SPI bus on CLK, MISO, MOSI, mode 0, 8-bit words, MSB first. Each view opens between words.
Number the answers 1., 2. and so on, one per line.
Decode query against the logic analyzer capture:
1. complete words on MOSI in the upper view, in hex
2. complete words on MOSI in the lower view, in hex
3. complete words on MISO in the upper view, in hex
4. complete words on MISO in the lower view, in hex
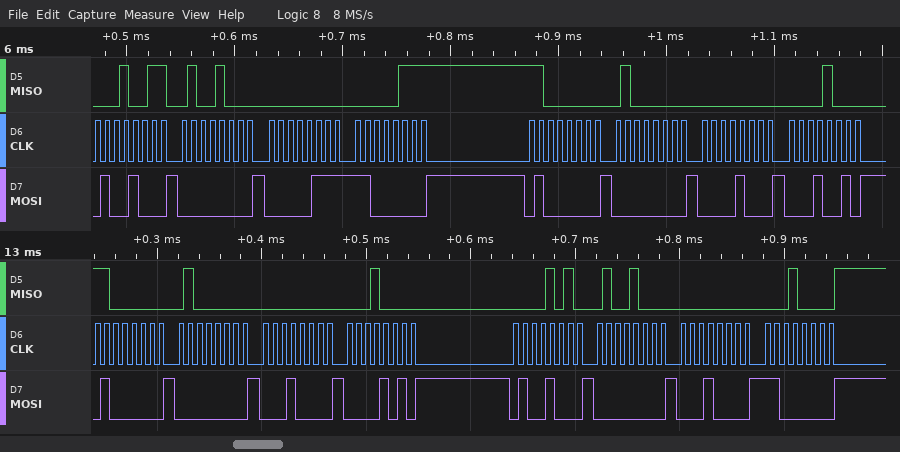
1. 48, 00, 07, C0, 40, 00, 08, 12
2. 40, 00, 10, 0A, 48, 00, 10, C0
3. 13, 48, 00, 07, C0, 40, 00, 08
4. C0, 40, 00, 10, 0A, 48, 00, 10
